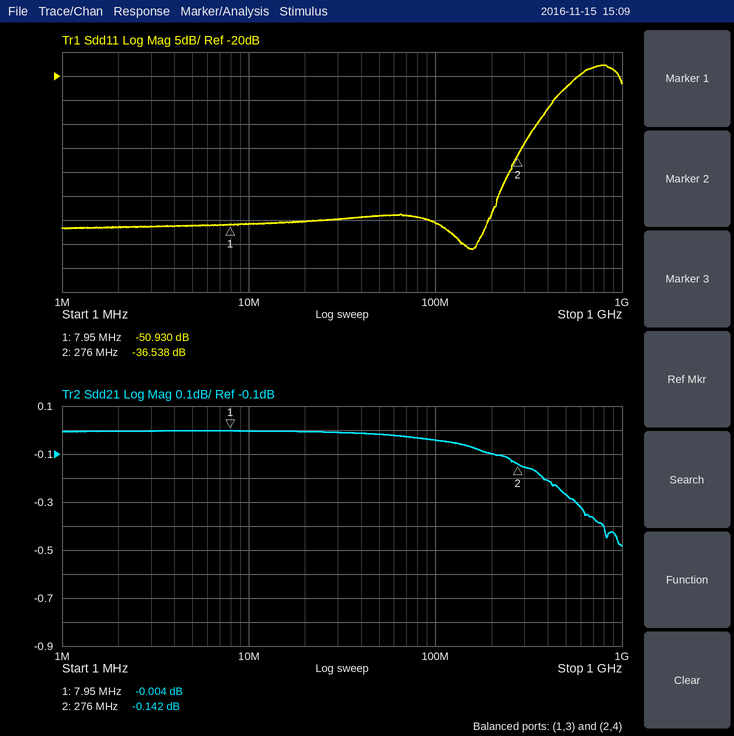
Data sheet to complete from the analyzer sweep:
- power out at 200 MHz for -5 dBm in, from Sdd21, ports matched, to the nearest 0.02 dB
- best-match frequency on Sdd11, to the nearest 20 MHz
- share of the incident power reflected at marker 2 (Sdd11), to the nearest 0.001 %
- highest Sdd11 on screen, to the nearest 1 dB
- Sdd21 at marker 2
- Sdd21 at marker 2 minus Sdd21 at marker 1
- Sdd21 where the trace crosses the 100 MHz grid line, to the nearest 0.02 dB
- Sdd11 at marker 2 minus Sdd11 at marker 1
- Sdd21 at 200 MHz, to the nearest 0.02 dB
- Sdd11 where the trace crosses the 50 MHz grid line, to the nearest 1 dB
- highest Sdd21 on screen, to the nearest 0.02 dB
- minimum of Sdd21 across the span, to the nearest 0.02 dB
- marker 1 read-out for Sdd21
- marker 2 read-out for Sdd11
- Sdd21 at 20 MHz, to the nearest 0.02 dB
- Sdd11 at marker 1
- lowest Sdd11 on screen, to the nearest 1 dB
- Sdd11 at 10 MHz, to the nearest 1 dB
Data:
-5.10 dBm
160 MHz
0.022 %
-18 dB
-0.142 dB
-0.138 dB
-0.04 dB
14.392 dB
-0.10 dB
-49 dB
0.00 dB
-0.48 dB
-0.004 dB
-36.538 dB
0.00 dB
-50.930 dB
-56 dB
-51 dB
